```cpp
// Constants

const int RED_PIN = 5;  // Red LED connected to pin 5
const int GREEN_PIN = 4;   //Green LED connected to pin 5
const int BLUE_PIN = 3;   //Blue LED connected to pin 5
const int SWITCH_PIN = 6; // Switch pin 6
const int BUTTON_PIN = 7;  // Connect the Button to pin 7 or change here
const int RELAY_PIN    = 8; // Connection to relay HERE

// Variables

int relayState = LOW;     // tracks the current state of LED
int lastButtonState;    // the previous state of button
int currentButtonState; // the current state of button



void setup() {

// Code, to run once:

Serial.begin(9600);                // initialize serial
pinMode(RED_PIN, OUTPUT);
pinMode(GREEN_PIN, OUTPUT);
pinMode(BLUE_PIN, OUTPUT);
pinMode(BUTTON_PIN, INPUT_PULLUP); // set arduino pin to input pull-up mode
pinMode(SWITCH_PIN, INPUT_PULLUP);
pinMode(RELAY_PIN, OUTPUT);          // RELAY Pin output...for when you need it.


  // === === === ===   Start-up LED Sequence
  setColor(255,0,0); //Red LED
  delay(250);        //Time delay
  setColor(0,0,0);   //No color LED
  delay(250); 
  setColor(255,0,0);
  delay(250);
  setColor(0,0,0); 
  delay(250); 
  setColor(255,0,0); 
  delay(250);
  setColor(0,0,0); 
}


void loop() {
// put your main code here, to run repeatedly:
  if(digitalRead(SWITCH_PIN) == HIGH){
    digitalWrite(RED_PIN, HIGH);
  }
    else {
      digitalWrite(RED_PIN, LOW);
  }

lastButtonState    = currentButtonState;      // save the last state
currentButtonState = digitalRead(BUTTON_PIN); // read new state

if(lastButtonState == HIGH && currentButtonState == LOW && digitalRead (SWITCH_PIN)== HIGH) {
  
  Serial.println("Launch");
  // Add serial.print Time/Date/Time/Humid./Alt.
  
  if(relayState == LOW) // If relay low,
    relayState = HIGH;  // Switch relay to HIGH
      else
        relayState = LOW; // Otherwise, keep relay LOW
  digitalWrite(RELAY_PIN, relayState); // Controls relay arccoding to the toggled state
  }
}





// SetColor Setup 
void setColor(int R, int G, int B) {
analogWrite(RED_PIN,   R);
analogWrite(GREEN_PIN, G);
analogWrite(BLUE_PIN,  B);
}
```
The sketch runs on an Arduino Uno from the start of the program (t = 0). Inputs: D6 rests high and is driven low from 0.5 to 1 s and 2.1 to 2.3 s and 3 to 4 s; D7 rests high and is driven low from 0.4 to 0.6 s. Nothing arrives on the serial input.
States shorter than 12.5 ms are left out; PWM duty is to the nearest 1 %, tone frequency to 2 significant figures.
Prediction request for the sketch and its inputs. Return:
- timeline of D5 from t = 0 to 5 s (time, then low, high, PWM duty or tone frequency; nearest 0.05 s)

0 s high; 0.25 s low; 0.5 s high; 0.75 s low; 1 s high; 2.1 s low; 2.3 s high; 3 s low; 4 s high
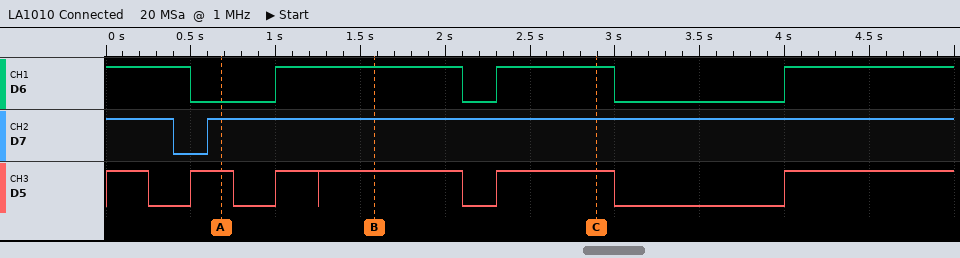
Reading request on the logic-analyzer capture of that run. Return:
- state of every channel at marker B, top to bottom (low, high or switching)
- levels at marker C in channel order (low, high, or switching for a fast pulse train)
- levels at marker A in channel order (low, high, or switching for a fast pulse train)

D6 high, D7 high, D5 high
D6 high, D7 high, D5 high
D6 low, D7 high, D5 high
